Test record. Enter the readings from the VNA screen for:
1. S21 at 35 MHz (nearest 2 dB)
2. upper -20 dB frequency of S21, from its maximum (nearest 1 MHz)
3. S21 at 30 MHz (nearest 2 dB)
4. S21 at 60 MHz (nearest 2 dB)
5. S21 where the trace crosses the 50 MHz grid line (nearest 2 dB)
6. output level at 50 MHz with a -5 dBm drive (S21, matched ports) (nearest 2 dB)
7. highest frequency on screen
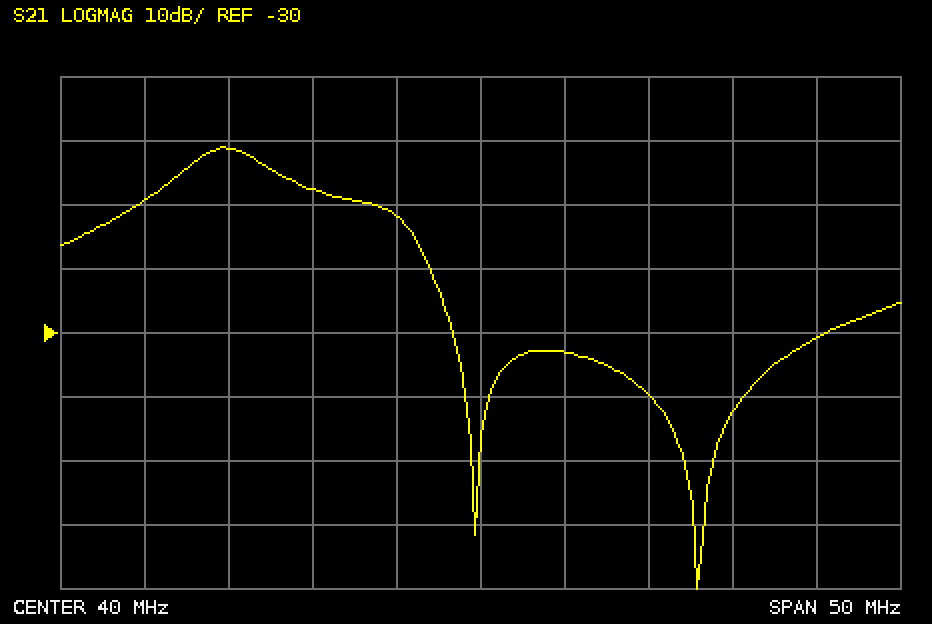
-12 dB
37 MHz
-8 dB
-30 dB
-40 dB
-44 dBm
65 MHz
